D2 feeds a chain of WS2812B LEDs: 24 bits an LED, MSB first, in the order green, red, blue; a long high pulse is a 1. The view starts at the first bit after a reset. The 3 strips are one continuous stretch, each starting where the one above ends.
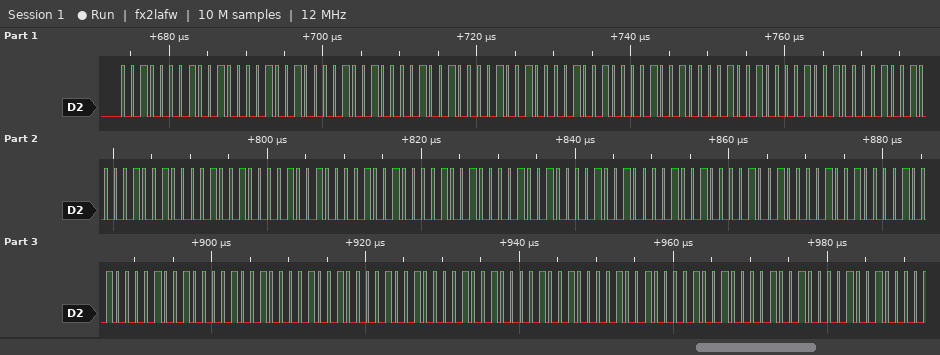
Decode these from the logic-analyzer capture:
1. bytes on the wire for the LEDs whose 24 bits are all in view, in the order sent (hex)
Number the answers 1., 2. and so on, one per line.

1. 21 21 21 21 21 21 21 21 21 21 21 21 21 21 21 21 21 21 21 21 21 21 21 21 21 21 21 21 21 21
